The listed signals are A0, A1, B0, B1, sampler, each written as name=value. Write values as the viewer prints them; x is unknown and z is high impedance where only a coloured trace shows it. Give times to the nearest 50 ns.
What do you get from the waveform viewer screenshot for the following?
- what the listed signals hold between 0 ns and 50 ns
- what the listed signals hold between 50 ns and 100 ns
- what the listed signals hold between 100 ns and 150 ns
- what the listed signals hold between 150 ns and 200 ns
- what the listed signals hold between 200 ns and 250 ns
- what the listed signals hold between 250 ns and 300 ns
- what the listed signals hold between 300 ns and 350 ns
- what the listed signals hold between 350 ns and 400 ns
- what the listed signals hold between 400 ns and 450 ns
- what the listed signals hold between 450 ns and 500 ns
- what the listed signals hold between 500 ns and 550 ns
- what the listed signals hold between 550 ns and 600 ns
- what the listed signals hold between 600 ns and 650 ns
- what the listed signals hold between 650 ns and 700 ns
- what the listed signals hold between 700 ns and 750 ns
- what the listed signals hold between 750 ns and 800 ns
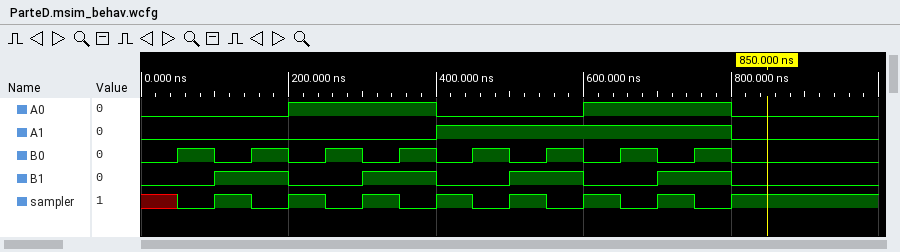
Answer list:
A0=0, A1=0, B0=0, B1=0, sampler=x
A0=0, A1=0, B0=1, B1=0, sampler=0
A0=0, A1=0, B0=0, B1=1, sampler=1
A0=0, A1=0, B0=1, B1=1, sampler=0
A0=1, A1=0, B0=0, B1=0, sampler=1
A0=1, A1=0, B0=1, B1=0, sampler=0
A0=1, A1=0, B0=0, B1=1, sampler=1
A0=1, A1=0, B0=1, B1=1, sampler=0
A0=0, A1=1, B0=0, B1=0, sampler=1
A0=0, A1=1, B0=1, B1=0, sampler=0
A0=0, A1=1, B0=0, B1=1, sampler=1
A0=0, A1=1, B0=1, B1=1, sampler=0
A0=1, A1=1, B0=0, B1=0, sampler=1
A0=1, A1=1, B0=1, B1=0, sampler=0
A0=1, A1=1, B0=0, B1=1, sampler=1
A0=1, A1=1, B0=1, B1=1, sampler=0
